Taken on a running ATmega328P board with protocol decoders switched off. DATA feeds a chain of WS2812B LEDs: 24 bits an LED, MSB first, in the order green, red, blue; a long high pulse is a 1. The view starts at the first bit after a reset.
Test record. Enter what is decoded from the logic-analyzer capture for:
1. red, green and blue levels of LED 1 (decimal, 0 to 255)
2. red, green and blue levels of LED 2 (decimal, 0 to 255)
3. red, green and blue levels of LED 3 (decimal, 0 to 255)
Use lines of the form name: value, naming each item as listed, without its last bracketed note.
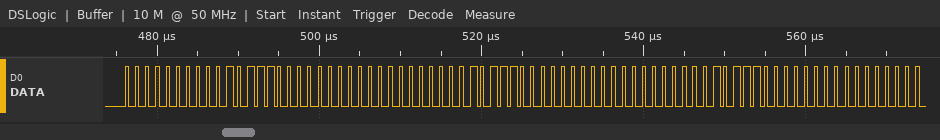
red, green and blue levels of LED 1: 46, 0, 0
red, green and blue levels of LED 2: 46, 0, 0
red, green and blue levels of LED 3: 46, 0, 0
